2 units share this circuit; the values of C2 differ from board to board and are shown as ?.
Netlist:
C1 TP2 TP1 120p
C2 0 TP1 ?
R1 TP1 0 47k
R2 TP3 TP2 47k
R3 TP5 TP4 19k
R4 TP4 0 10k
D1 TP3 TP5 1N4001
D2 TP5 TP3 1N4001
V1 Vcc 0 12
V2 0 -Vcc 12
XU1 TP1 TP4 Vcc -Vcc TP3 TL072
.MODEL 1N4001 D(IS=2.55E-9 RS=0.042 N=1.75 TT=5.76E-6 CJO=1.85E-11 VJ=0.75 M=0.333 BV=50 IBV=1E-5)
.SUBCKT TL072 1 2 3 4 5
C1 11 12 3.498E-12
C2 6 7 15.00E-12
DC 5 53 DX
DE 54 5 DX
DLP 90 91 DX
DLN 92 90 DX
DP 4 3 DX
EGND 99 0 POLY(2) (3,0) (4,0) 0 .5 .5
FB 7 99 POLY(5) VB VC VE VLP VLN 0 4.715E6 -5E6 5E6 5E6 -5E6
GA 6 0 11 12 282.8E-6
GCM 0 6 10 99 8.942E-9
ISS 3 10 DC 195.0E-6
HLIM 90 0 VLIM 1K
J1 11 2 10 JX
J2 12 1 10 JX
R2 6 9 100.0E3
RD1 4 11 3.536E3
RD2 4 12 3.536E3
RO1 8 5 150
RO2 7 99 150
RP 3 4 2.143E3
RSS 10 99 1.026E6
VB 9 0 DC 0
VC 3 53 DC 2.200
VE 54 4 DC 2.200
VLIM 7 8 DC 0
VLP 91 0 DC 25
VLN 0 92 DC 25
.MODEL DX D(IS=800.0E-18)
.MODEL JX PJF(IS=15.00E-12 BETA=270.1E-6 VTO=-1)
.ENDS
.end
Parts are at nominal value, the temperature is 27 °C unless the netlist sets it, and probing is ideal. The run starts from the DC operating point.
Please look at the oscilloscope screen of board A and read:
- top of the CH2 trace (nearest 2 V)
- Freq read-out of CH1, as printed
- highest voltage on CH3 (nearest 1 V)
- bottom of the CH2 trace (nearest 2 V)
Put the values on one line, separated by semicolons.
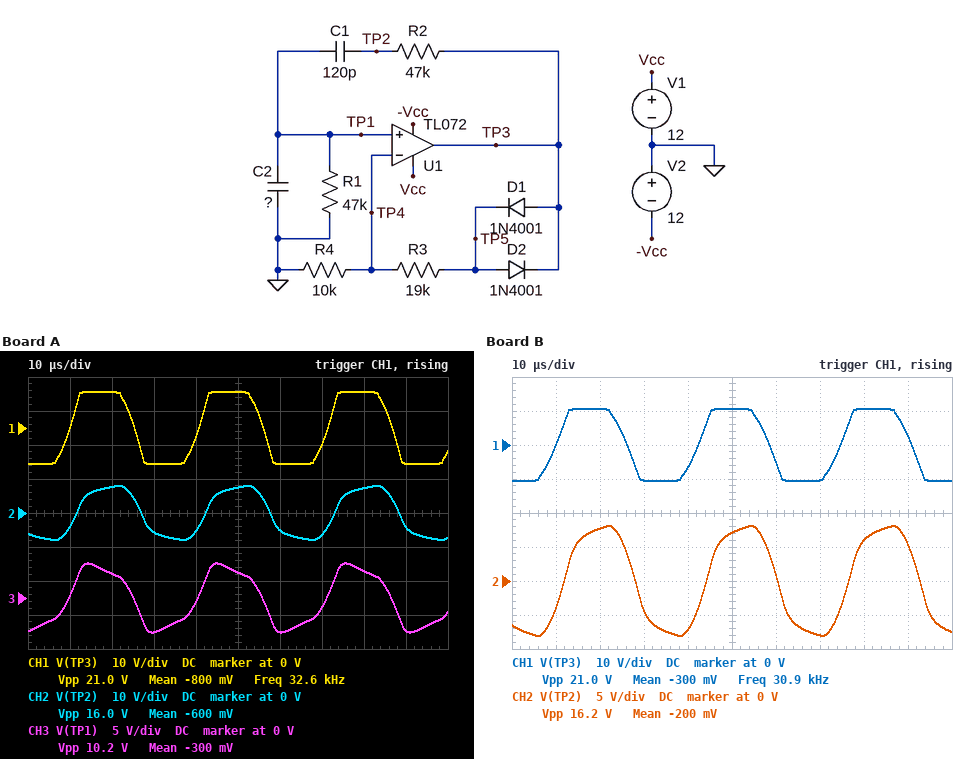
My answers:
8 V; 32.6 kHz; 5 V; -8 V
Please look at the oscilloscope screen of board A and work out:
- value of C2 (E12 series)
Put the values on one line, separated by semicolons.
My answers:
56 pF
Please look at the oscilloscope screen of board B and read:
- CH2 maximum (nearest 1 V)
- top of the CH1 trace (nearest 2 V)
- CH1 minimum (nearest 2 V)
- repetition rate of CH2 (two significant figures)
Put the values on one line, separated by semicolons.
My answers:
8 V; 10 V; -10 V; 31 kHz
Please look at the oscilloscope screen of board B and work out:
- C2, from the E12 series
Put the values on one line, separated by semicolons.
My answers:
68 pF
